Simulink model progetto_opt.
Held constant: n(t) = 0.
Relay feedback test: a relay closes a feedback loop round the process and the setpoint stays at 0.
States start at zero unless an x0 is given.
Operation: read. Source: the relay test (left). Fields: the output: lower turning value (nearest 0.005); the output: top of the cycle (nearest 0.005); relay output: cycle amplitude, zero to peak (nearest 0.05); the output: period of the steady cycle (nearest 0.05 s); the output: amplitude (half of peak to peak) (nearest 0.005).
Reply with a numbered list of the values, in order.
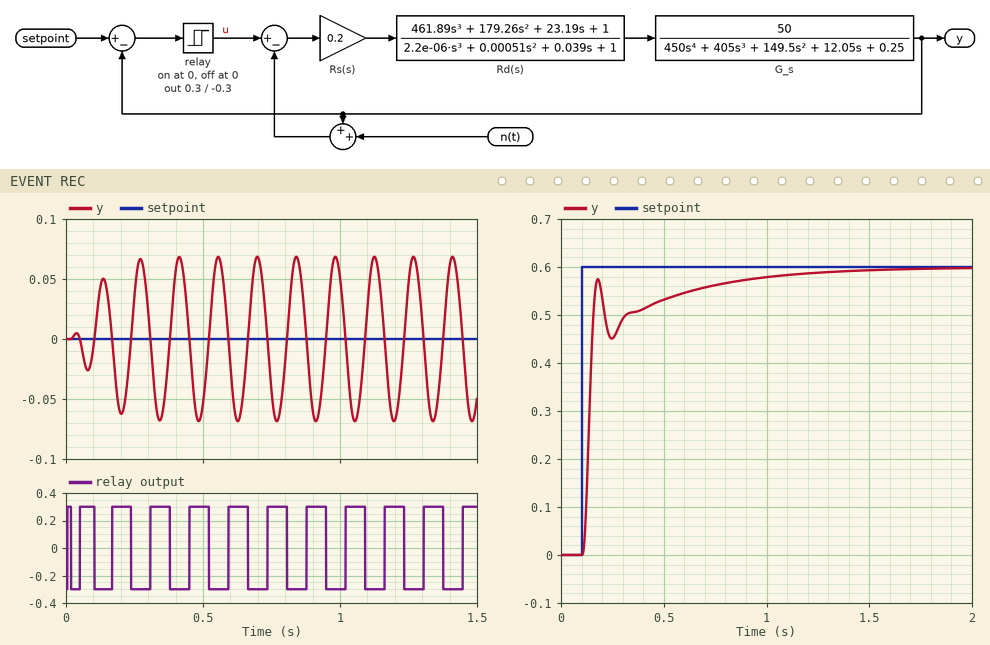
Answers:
1. -0.070
2. 0.070
3. 0.30
4. 0.15 s
5. 0.070
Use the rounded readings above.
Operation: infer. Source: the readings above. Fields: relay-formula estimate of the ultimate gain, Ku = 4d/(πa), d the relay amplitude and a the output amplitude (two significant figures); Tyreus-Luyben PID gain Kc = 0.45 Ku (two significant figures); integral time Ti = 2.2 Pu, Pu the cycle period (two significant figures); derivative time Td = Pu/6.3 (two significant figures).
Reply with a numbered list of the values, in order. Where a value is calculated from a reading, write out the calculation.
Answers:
1. 4 × 0.3 / (π × 0.07) = 5.5
2. 0.45 × 5.5 = 2.5
3. 2.2 × 0.15 = 0.33 s
4. 0.15 / 6.3 = 0.024 s
